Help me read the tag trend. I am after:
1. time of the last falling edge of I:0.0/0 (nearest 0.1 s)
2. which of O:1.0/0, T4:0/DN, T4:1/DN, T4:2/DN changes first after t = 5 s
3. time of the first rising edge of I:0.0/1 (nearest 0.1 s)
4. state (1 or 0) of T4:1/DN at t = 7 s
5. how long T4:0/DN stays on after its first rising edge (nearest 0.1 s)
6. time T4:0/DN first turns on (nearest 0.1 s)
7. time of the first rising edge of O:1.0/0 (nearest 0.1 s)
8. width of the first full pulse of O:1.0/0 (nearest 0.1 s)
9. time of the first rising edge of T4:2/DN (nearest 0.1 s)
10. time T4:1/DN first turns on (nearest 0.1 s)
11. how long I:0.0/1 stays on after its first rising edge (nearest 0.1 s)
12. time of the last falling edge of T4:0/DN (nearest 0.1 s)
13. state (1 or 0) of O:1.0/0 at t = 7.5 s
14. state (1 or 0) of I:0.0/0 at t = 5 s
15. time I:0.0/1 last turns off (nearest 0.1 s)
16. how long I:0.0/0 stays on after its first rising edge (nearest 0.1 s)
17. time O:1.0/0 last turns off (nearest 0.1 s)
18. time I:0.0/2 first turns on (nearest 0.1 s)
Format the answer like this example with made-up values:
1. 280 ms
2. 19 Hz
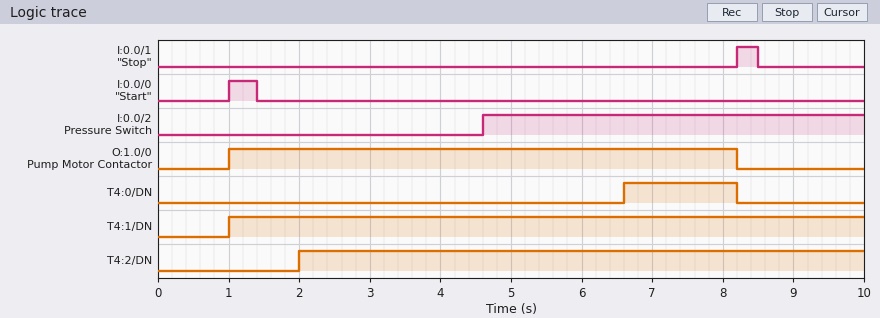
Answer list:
1. 1.4 s
2. T4:0/DN
3. 8.2 s
4. 1
5. 1.6 s
6. 6.6 s
7. 1.0 s
8. 7.2 s
9. 2.0 s
10. 1.0 s
11. 0.3 s
12. 8.2 s
13. 1
14. 0
15. 8.5 s
16. 0.4 s
17. 8.2 s
18. 4.6 s
